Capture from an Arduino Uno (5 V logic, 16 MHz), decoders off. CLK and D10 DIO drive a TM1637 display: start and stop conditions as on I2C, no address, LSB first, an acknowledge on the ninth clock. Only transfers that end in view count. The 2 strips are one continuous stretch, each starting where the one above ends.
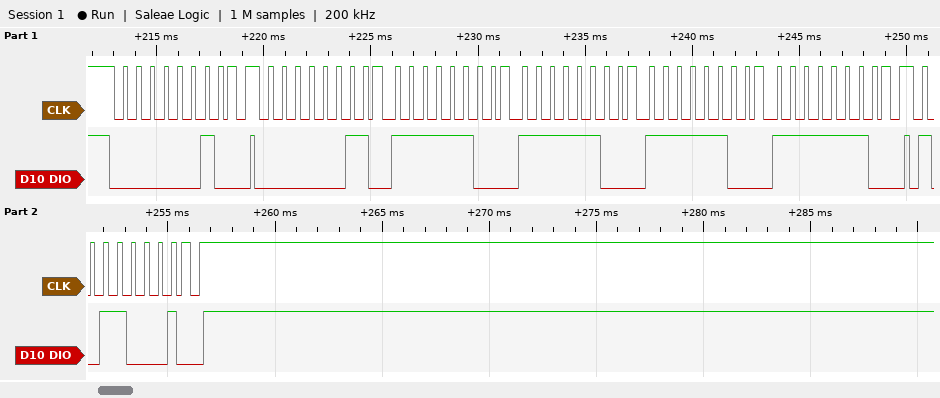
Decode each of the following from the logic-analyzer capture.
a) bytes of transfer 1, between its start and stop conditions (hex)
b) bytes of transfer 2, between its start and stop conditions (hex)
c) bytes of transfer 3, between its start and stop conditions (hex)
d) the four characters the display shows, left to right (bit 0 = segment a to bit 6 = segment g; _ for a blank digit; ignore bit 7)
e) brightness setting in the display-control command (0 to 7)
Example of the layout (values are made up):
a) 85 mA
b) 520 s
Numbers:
a) 40
b) C0 3F 3F 3F 7F
c) 8D
d) 0008
e) 5
